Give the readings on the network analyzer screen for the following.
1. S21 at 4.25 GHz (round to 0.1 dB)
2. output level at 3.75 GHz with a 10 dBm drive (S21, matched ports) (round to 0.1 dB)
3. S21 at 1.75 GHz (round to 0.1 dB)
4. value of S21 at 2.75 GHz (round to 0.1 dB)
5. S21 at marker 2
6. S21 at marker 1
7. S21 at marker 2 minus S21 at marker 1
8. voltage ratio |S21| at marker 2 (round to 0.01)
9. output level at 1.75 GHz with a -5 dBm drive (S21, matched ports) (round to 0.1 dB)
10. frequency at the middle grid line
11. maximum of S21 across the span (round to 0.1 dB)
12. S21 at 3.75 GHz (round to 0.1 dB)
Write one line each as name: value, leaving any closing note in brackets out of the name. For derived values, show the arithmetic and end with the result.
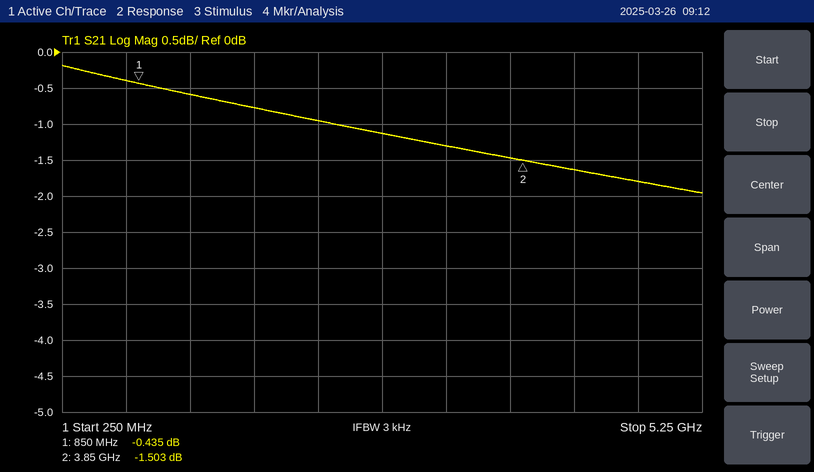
S21 at 4.25 GHz: -1.6 dB
output level at 3.75 GHz with a 10 dBm drive (S21, matched ports): 10 dBm + (-1.5 dB) = 8.5 dBm
S21 at 1.75 GHz: -0.8 dB
value of S21 at 2.75 GHz: -1.1 dB
S21 at marker 2: -1.503 dB
S21 at marker 1: -0.435 dB
S21 at marker 2 minus S21 at marker 1: -1.503 − (-0.435) = -1.068 dB
voltage ratio |S21| at marker 2: 10^(-1.503/20) ≈ 0.84
output level at 1.75 GHz with a -5 dBm drive (S21, matched ports): -5 dBm + (-0.8 dB) = -5.8 dBm
frequency at the middle grid line: 2.75 GHz
maximum of S21 across the span: -0.2 dB
S21 at 3.75 GHz: -1.5 dB
